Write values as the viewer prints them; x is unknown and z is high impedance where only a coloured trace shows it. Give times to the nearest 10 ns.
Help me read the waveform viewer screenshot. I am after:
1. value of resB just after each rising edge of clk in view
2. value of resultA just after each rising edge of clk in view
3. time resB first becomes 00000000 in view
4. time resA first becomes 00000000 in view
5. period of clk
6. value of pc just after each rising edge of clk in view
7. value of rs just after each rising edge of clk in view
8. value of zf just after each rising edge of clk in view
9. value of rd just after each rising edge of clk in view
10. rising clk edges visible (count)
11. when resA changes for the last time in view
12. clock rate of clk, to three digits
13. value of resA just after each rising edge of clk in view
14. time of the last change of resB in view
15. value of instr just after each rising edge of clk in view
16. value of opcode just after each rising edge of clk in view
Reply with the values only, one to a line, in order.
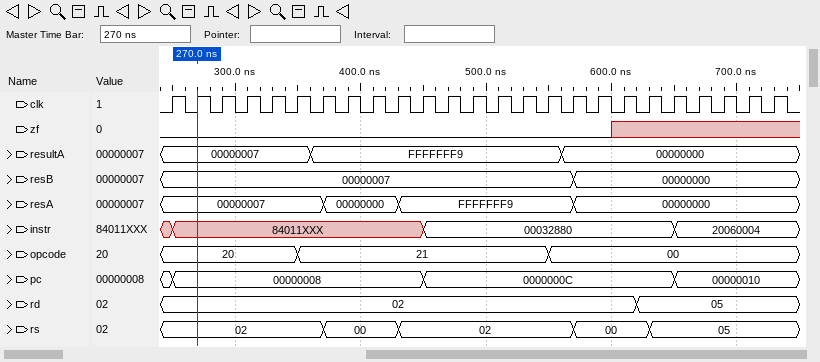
00000007, 00000007, 00000007, 00000007, 00000007, 00000007, 00000007, 00000007, 00000007, 00000007, 00000007, 00000007, 00000007, 00000007, 00000007, 00000007, 00000000, 00000000, 00000000, 00000000, 00000000, 00000000, 00000000, 00000000, 00000000
00000007, 00000007, 00000007, 00000007, 00000007, 00000007, FFFFFFF9, FFFFFFF9, FFFFFFF9, FFFFFFF9, FFFFFFF9, FFFFFFF9, FFFFFFF9, FFFFFFF9, FFFFFFF9, FFFFFFF9, 00000000, 00000000, 00000000, 00000000, 00000000, 00000000, 00000000, 00000000, 00000000
570 ns
370 ns
20 ns
00000008, 00000008, 00000008, 00000008, 00000008, 00000008, 00000008, 00000008, 00000008, 00000008, 0000000C, 0000000C, 0000000C, 0000000C, 0000000C, 0000000C, 0000000C, 0000000C, 0000000C, 0000000C, 00000010, 00000010, 00000010, 00000010, 00000010
02, 02, 02, 02, 02, 02, 00, 00, 00, 02, 02, 02, 02, 02, 02, 02, 00, 00, 00, 05, 05, 05, 05, 05, 05
0 0 0 0 0 0 0 0 0 0 0 0 0 0 0 0 0 0 x x x x x x x
02, 02, 02, 02, 02, 02, 02, 02, 02, 02, 02, 02, 02, 02, 02, 02, 02, 02, 02, 05, 05, 05, 05, 05, 05
25
570 ns
50.0 MHz
00000007, 00000007, 00000007, 00000007, 00000007, 00000007, 00000000, 00000000, 00000000, FFFFFFF9, FFFFFFF9, FFFFFFF9, FFFFFFF9, FFFFFFF9, FFFFFFF9, FFFFFFF9, 00000000, 00000000, 00000000, 00000000, 00000000, 00000000, 00000000, 00000000, 00000000
570 ns
84011XXX, 84011XXX, 84011XXX, 84011XXX, 84011XXX, 84011XXX, 84011XXX, 84011XXX, 84011XXX, 84011XXX, 00032880, 00032880, 00032880, 00032880, 00032880, 00032880, 00032880, 00032880, 00032880, 00032880, 20060004, 20060004, 20060004, 20060004, 20060004
20, 20, 20, 20, 20, 21, 21, 21, 21, 21, 21, 21, 21, 21, 21, 00, 00, 00, 00, 00, 00, 00, 00, 00, 00
